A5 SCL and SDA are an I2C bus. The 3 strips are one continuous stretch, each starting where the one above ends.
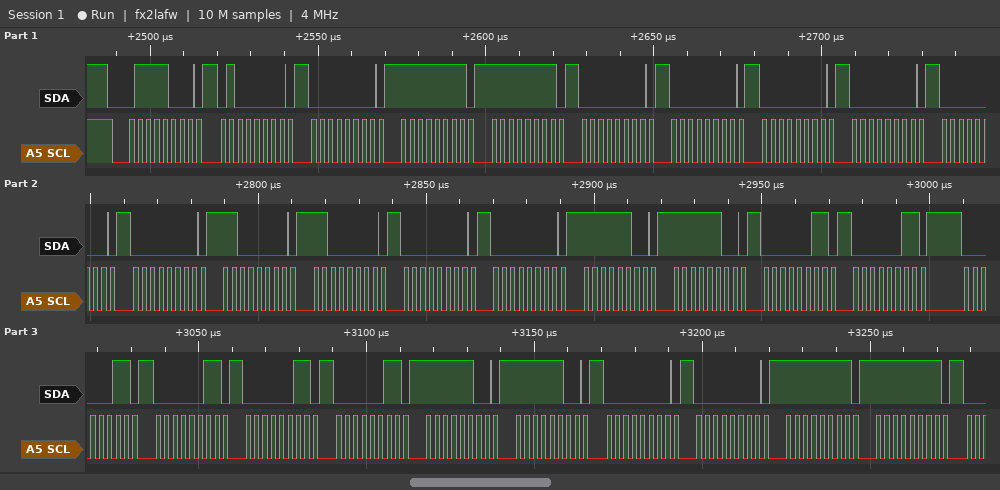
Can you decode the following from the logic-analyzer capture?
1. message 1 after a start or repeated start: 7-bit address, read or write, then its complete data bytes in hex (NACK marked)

0x3C write: 40 00 FF FF 00 00 00 00 00 00 C0 C0 00 00 FC FC 03 03 03 03 03 03 FC FC 00 00 FF FF
